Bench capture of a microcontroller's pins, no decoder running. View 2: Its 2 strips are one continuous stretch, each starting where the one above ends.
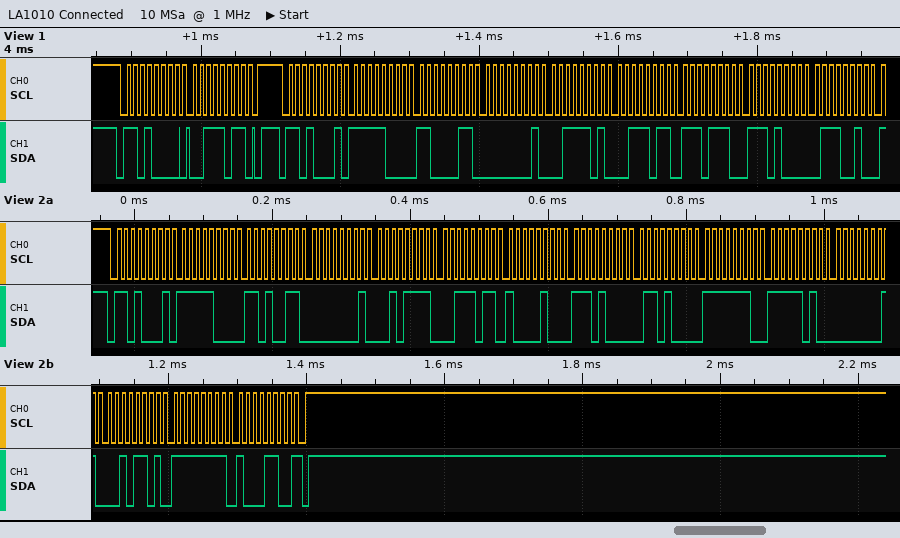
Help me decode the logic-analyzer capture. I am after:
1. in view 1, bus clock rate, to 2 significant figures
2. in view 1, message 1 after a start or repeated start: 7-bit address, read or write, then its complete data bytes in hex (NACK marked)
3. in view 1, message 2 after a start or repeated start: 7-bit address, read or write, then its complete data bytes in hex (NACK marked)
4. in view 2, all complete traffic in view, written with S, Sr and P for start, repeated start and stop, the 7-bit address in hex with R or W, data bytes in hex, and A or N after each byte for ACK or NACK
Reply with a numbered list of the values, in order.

1. 100 kHz
2. 0x68 write: 3B
3. 0x68 read: F8 C3 01 3D 3B EE E8 72
4. S 68R A F8 A D3 A 01 A 2F A 3B A 84 A E8 A 68 A FE A FA A 01 A 2D A FF A 8C N P
